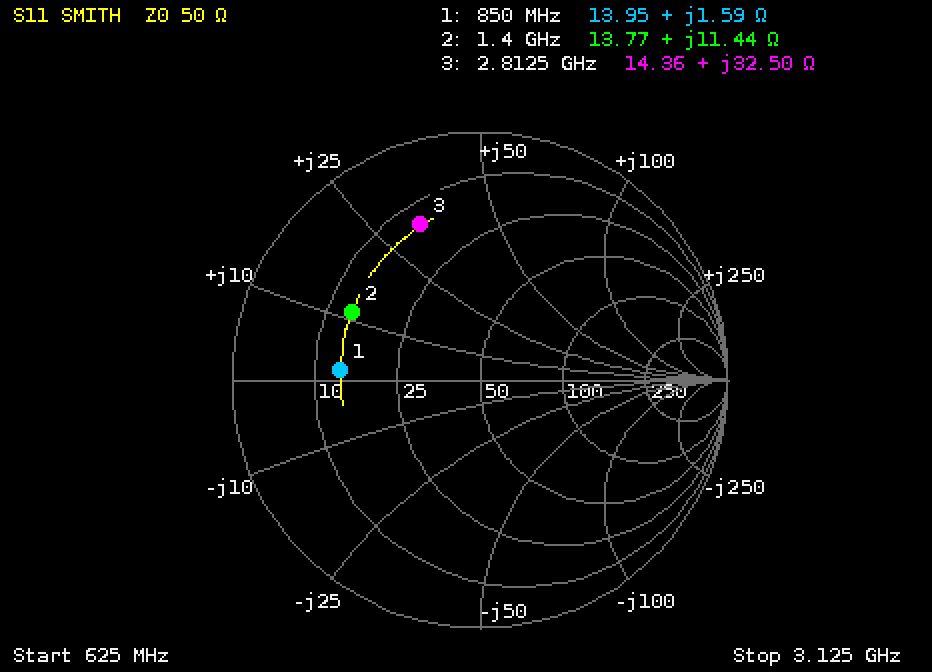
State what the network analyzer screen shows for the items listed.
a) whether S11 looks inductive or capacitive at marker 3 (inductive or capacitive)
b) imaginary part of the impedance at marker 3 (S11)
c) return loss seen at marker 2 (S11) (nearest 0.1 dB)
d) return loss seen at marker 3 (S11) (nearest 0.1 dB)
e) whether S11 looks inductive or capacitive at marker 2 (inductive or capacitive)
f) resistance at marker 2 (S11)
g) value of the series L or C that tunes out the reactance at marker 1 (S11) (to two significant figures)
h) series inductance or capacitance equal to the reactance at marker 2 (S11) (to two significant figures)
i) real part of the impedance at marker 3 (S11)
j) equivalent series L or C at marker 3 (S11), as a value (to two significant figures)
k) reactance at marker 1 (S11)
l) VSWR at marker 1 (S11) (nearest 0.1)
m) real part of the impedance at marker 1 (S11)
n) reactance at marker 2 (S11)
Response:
inductive
+32.50 Ω
4.6 dB
3.5 dB
inductive
13.77 Ω
120 pF
1.3 nH
14.36 Ω
1.8 nH
+1.59 Ω
3.6
13.95 Ω
+11.44 Ω
